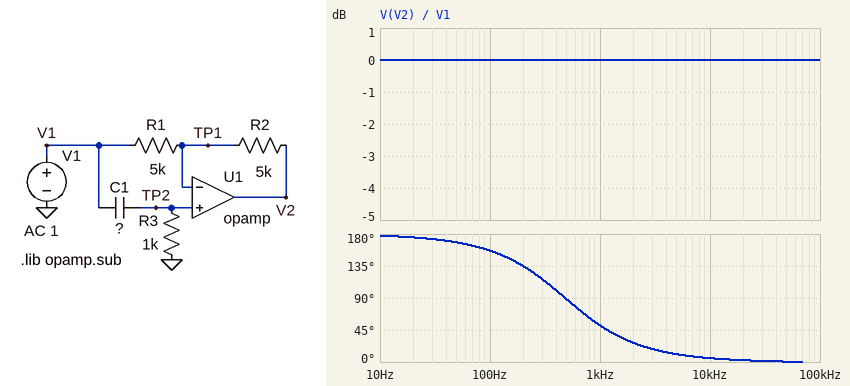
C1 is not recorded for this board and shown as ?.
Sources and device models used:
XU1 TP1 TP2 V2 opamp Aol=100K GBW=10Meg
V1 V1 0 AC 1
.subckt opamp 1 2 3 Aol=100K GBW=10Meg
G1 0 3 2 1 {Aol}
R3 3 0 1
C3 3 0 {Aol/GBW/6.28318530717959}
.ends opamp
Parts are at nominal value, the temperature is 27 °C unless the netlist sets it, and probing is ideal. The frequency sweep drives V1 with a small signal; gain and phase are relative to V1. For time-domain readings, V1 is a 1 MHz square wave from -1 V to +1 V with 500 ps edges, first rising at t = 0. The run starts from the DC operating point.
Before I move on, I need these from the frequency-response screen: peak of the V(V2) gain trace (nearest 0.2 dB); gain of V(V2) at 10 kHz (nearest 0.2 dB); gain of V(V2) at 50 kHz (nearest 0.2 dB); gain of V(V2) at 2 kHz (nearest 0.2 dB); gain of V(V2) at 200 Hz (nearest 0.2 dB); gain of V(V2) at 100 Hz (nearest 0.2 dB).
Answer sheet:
0 dB
0 dB
0 dB
0 dB
0 dB
0 dB
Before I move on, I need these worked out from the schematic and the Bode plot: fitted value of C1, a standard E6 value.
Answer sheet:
330 nF
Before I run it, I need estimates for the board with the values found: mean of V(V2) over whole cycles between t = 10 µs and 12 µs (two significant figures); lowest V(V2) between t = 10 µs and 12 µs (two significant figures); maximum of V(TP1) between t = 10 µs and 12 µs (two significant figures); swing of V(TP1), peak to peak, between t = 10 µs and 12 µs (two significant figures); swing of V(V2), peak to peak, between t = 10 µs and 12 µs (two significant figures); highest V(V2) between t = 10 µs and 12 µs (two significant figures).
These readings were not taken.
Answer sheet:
1.9 V
930 mV
2.0 V
2.0 V
2.0 V
2.9 V
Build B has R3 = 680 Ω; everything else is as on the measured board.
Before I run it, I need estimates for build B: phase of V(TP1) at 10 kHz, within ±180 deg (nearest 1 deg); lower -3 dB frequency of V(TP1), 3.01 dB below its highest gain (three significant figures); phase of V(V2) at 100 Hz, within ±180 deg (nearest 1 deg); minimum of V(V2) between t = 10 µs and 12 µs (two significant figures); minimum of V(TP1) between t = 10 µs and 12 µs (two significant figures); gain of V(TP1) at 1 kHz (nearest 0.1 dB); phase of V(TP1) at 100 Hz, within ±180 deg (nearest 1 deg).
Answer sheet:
4 deg
709 Hz
164 deg
900 mV
-52 mV
-1.8 dB
82 deg
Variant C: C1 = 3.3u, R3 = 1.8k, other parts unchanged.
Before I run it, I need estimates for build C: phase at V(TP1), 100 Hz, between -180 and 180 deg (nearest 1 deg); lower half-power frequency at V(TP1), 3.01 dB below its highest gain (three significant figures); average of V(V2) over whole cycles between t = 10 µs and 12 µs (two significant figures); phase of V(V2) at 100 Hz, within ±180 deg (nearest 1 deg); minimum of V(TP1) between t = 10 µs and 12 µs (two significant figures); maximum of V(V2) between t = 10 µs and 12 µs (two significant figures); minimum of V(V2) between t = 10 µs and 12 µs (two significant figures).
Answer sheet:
15 deg
26.8 Hz
2.0 V
30 deg
-2.0 mV
3.0 V
1.0 V
